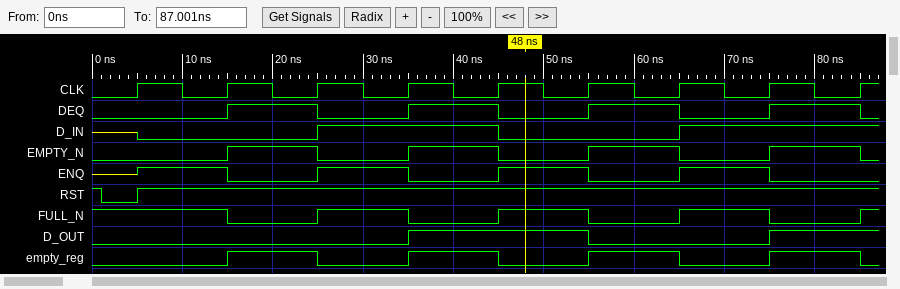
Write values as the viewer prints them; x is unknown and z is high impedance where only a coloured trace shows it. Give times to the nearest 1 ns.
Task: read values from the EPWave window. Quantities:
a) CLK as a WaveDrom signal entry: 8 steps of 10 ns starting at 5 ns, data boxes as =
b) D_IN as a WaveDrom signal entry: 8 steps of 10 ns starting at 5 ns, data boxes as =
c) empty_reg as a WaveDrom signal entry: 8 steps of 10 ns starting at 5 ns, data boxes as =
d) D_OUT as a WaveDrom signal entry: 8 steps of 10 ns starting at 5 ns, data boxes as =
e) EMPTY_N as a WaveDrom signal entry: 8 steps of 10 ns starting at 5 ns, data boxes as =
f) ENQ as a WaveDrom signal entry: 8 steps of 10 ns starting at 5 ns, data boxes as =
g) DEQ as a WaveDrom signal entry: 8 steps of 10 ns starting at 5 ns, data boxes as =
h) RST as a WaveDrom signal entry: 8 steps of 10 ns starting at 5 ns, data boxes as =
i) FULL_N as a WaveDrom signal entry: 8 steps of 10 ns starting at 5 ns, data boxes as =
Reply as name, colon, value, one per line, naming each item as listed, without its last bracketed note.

CLK as a WaveDrom signal entry: 8 steps of 10 ns starting at 5 ns, data boxes as =: {name: 'CLK', wave: 'p.......'}
D_IN as a WaveDrom signal entry: 8 steps of 10 ns starting at 5 ns, data boxes as =: {name: 'D_IN', wave: '0.1.0.1.'}
empty_reg as a WaveDrom signal entry: 8 steps of 10 ns starting at 5 ns, data boxes as =: {name: 'empty_reg', wave: '01010101'}
D_OUT as a WaveDrom signal entry: 8 steps of 10 ns starting at 5 ns, data boxes as =: {name: 'D_OUT', wave: '0..1.0.1'}
EMPTY_N as a WaveDrom signal entry: 8 steps of 10 ns starting at 5 ns, data boxes as =: {name: 'EMPTY_N', wave: '01010101'}
ENQ as a WaveDrom signal entry: 8 steps of 10 ns starting at 5 ns, data boxes as =: {name: 'ENQ', wave: '10101010'}
DEQ as a WaveDrom signal entry: 8 steps of 10 ns starting at 5 ns, data boxes as =: {name: 'DEQ', wave: '01010101'}
RST as a WaveDrom signal entry: 8 steps of 10 ns starting at 5 ns, data boxes as =: {name: 'RST', wave: '1.......'}
FULL_N as a WaveDrom signal entry: 8 steps of 10 ns starting at 5 ns, data boxes as =: {name: 'FULL_N', wave: '10101010'}
